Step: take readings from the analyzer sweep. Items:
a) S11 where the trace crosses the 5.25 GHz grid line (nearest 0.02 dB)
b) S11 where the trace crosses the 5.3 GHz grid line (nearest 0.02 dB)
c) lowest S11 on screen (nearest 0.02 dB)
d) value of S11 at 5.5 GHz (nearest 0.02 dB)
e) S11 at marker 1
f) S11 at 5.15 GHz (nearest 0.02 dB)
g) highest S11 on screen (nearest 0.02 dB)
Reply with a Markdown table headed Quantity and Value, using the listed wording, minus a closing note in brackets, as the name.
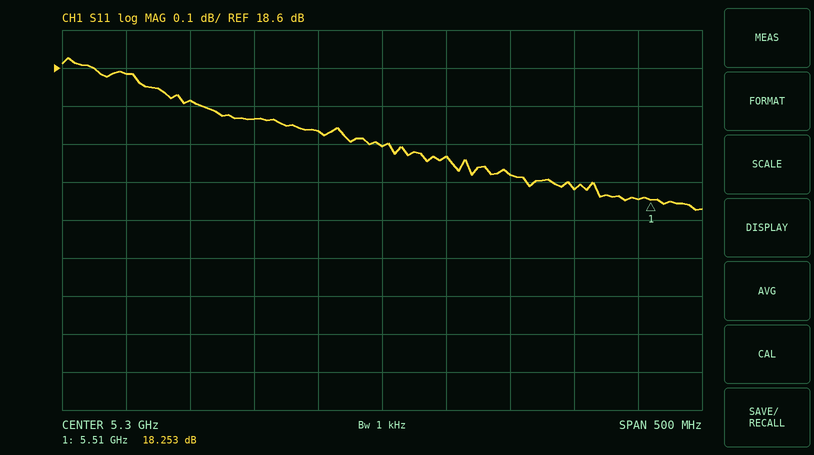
| Quantity | Value |
|---|---|
| S11 where the trace crosses the 5.25 GHz grid line | 18.44 dB |
| S11 where the trace crosses the 5.3 GHz grid line | 18.40 dB |
| lowest S11 on screen | 18.22 dB |
| value of S11 at 5.5 GHz | 18.26 dB |
| S11 at marker 1 | 18.253 dB |
| S11 at 5.15 GHz | 18.52 dB |
| highest S11 on screen | 18.62 dB |
